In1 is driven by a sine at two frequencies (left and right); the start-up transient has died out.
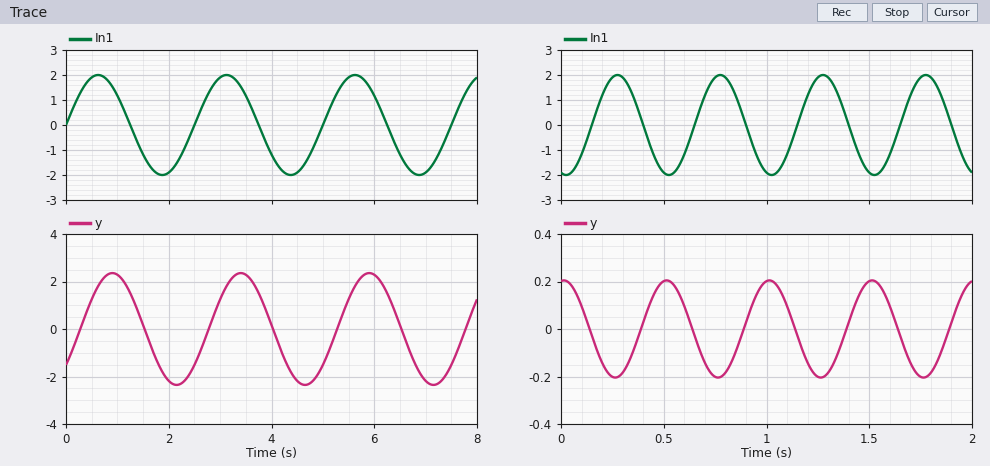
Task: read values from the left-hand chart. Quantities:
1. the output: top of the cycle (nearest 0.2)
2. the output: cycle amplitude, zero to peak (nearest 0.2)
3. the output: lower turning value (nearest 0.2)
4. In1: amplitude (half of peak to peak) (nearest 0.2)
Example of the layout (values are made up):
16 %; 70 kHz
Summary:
2.4; 2.4; -2.4; 2.0
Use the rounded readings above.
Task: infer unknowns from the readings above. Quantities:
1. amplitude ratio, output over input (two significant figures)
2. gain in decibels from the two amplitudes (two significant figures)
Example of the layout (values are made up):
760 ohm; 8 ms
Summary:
1.2; 1.6 dB
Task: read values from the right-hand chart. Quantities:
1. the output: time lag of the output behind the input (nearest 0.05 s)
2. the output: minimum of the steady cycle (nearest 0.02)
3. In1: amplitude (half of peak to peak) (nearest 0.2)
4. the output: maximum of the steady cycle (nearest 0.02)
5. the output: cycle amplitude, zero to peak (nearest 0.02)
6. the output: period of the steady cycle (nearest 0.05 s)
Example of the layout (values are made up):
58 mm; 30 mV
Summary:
0.25 s; -0.20; 2.0; 0.20; 0.20; 0.50 s
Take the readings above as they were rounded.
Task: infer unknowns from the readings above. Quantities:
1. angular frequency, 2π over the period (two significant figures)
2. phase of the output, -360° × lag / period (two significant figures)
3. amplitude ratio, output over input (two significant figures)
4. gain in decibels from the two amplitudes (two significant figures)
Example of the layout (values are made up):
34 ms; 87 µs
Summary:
13 rad/s; -180°; 0.10; -20 dB
